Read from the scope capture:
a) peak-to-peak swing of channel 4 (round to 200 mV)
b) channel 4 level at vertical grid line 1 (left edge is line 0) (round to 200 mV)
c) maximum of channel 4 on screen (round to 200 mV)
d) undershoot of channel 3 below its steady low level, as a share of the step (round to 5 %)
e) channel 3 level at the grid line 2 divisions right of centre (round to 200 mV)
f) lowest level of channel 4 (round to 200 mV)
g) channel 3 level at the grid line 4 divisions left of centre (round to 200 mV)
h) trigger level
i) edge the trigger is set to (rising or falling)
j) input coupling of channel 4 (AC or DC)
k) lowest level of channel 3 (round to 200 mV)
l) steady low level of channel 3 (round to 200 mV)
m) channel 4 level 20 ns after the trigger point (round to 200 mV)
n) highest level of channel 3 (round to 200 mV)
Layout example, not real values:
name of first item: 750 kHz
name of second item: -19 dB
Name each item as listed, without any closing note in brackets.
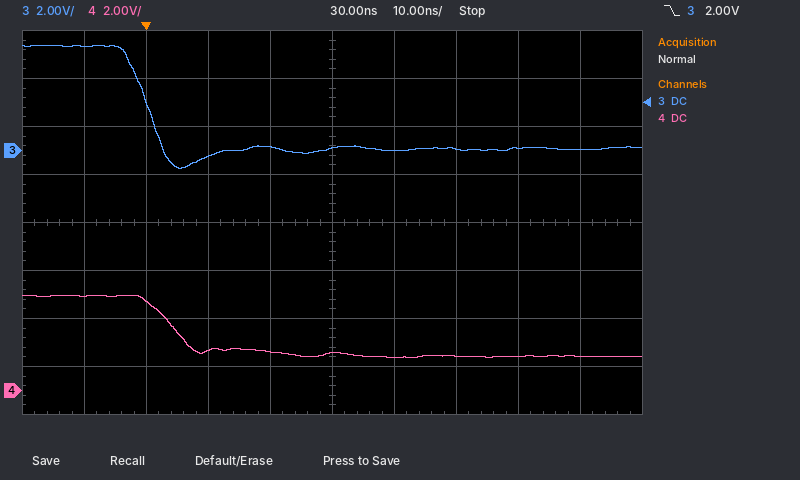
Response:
peak-to-peak swing of channel 4: 2.6 V
channel 4 level at vertical grid line 1 (left edge is line 0): 4.0 V
maximum of channel 4 on screen: 4.0 V
undershoot of channel 3 below its steady low level, as a share of the step: 20 %
channel 3 level at the grid line 2 divisions right of centre: 0.0 V
lowest level of channel 4: 1.4 V
channel 3 level at the grid line 4 divisions left of centre: 4.4 V
trigger level: 2.00 V
edge the trigger is set to: falling
input coupling of channel 4: DC
lowest level of channel 3: -800 mV
steady low level of channel 3: 0.0 V
channel 4 level 20 ns after the trigger point: 1.6 V
highest level of channel 3: 4.4 V
